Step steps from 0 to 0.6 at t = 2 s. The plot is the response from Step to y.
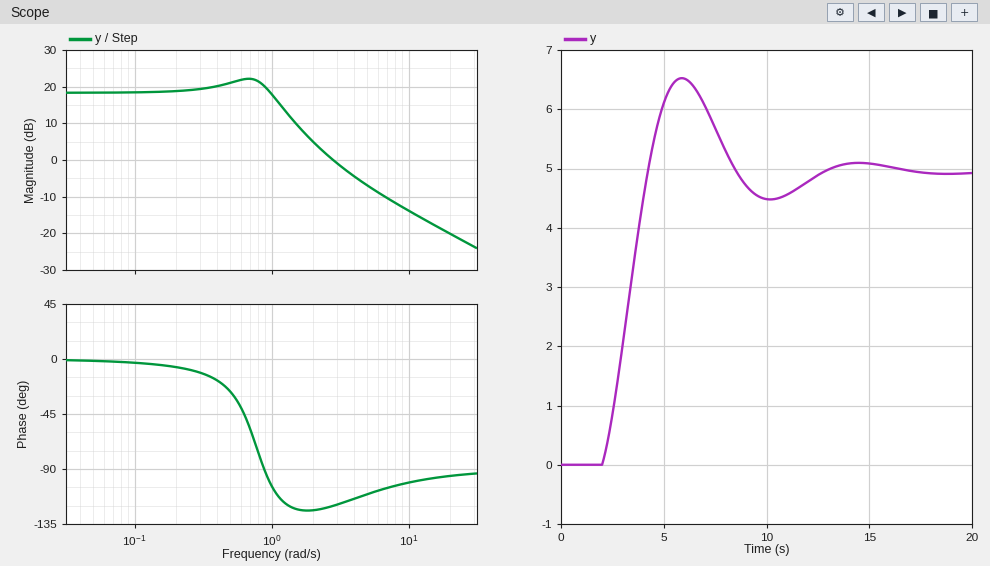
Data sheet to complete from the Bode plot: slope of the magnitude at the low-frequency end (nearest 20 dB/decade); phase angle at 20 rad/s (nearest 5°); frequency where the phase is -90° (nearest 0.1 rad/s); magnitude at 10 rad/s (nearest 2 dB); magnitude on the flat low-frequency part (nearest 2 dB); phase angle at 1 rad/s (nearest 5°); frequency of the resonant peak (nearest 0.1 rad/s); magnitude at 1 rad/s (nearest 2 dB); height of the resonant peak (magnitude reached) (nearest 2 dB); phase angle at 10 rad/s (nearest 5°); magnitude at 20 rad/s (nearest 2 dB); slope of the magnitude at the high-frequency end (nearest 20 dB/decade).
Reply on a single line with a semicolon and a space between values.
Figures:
0 dB/decade; -95°; 0.9 rad/s; -14 dB; 18 dB; -105°; 0.7 rad/s; 18 dB; 22 dB; -100°; -20 dB; -20 dB/decade
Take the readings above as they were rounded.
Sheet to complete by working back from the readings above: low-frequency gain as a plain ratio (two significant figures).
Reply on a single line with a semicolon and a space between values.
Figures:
7.9
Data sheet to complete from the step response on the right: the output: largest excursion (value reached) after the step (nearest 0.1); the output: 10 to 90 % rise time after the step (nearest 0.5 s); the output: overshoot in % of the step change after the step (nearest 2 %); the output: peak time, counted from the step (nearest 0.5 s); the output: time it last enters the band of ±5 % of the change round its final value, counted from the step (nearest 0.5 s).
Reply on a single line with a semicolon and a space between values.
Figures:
6.5; 1.5 s; 32 %; 4.0 s; 9.5 s
